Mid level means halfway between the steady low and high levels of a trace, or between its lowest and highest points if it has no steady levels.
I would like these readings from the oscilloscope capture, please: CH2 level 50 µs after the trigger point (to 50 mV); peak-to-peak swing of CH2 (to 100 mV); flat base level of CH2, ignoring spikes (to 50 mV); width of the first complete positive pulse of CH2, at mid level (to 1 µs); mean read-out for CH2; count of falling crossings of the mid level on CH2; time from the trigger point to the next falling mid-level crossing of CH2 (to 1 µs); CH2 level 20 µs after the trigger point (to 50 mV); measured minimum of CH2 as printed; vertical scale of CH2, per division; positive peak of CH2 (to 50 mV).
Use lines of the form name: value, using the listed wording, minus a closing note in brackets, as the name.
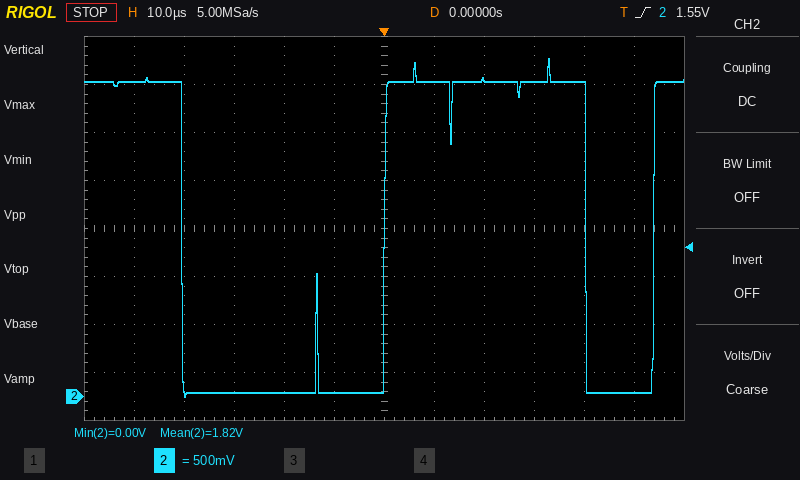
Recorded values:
CH2 level 50 µs after the trigger point: 50 mV
peak-to-peak swing of CH2: 3.50 V
flat base level of CH2, ignoring spikes: 50 mV
width of the first complete positive pulse of CH2, at mid level: 40 µs
mean read-out for CH2: 1.82 V
count of falling crossings of the mid level on CH2: 2
time from the trigger point to the next falling mid-level crossing of CH2: 40 µs
CH2 level 20 µs after the trigger point: 3.30 V
measured minimum of CH2 as printed: 0.00 V
vertical scale of CH2, per division: 500 mV
positive peak of CH2: 3.50 V
